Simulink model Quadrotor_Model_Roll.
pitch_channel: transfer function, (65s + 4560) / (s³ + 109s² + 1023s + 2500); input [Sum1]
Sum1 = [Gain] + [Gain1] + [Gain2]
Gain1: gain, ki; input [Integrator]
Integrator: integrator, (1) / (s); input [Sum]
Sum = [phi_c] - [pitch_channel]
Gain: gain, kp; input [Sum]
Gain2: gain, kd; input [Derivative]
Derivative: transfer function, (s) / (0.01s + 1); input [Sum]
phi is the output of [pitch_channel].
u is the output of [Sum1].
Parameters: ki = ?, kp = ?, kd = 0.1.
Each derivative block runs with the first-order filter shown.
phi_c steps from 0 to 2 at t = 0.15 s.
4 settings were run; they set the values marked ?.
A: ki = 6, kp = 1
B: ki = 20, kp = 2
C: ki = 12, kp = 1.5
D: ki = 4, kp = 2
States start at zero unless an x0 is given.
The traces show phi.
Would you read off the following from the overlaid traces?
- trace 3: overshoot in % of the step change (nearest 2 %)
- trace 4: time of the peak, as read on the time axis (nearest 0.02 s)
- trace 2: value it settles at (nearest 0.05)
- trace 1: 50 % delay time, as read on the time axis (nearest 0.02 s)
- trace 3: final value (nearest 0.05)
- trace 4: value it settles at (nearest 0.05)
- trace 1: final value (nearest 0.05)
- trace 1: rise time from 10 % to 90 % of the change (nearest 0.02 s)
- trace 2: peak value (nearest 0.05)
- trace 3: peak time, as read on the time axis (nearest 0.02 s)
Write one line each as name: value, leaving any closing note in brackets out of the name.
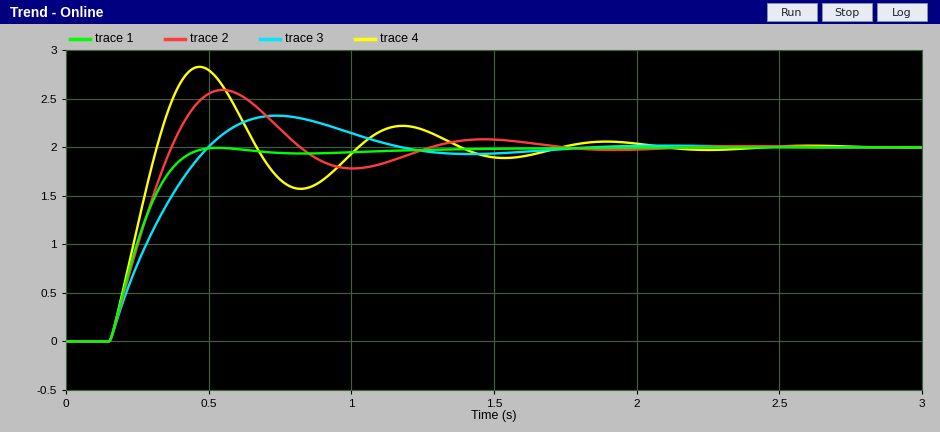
trace 3: overshoot in % of the step change: 16 %
trace 4: time of the peak, as read on the time axis: 0.46 s
trace 2: value it settles at: 2.00
trace 1: 50 % delay time, as read on the time axis: 0.24 s
trace 3: final value: 2.00
trace 4: value it settles at: 2.00
trace 1: final value: 2.00
trace 1: rise time from 10 % to 90 % of the change: 0.20 s
trace 2: peak value: 2.60
trace 3: peak time, as read on the time axis: 0.74 s
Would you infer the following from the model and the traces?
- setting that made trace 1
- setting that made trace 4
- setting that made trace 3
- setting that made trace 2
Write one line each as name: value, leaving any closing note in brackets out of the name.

setting that made trace 1: D
setting that made trace 4: B
setting that made trace 3: A
setting that made trace 2: C
